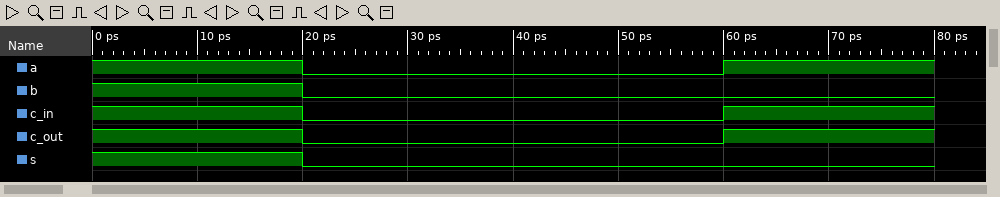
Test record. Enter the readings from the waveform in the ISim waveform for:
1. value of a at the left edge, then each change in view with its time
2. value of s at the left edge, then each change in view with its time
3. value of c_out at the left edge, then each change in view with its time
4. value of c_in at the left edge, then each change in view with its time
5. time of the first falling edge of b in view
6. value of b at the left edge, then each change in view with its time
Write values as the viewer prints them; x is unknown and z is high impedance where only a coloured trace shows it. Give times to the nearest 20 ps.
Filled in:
1, 0 at 20 ps, 1 at 60 ps
1, 0 at 20 ps
1, 0 at 20 ps, 1 at 60 ps
1, 0 at 20 ps, 1 at 60 ps
20 ps
1, 0 at 20 ps
